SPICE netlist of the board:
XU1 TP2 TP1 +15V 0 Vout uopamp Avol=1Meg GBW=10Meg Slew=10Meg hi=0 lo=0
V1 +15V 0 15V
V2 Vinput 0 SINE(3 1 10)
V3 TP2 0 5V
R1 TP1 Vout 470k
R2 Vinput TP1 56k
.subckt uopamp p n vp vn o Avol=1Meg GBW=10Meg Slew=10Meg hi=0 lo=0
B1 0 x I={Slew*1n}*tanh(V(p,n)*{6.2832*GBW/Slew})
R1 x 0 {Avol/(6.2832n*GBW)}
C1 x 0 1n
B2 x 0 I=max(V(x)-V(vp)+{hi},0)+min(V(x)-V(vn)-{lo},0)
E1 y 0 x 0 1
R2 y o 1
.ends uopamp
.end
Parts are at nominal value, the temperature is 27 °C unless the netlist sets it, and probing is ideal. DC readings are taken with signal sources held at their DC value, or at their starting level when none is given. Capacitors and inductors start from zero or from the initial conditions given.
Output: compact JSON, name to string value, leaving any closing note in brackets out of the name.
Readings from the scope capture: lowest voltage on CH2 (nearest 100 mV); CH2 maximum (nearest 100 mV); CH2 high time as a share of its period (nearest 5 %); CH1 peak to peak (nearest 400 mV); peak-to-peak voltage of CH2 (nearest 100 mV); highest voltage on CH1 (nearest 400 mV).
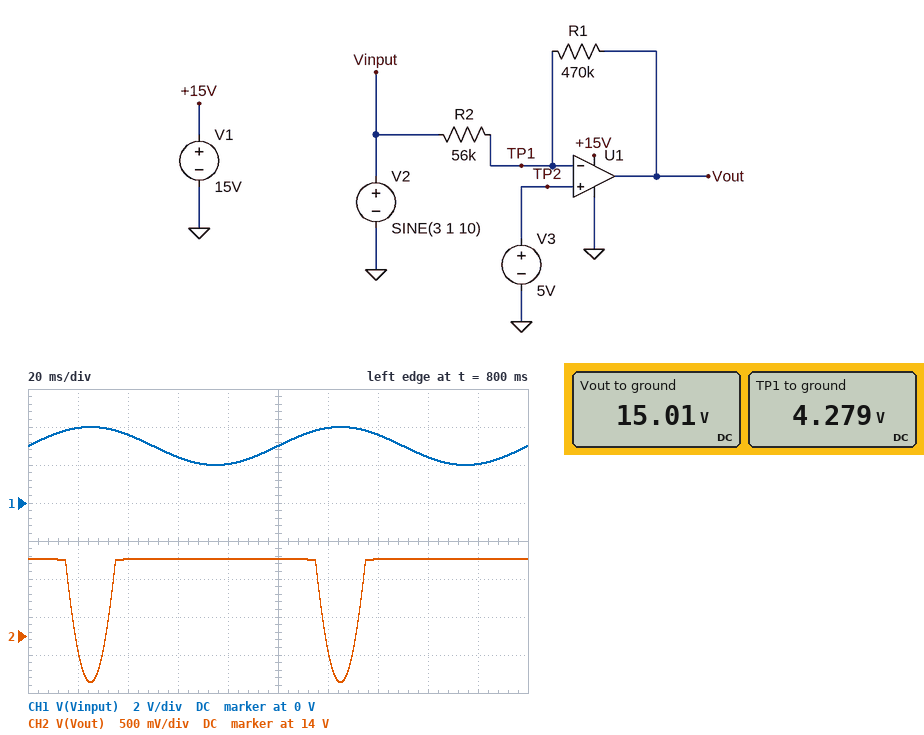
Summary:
{"lowest voltage on CH2": "13.4 V", "CH2 maximum": "15.0 V", "CH2 high time as a share of its period": "85 %", "CH1 peak to peak": "2.0 V", "peak-to-peak voltage of CH2": "1.6 V", "highest voltage on CH1": "4.0 V"}
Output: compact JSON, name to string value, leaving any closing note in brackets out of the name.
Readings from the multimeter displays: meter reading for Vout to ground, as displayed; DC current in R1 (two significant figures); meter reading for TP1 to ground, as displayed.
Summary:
{"meter reading for Vout to ground, as displayed": "15.01 V", "DC current in R1": "23 µA", "meter reading for TP1 to ground, as displayed": "4.279 V"}
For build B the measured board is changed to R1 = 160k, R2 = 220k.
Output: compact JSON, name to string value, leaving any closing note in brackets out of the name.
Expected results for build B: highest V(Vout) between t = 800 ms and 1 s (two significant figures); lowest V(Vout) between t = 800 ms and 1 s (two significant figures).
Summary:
{"highest V(Vout) between t = 800 ms and 1 s": "7.2 V", "lowest V(Vout) between t = 800 ms and 1 s": "5.7 V"}
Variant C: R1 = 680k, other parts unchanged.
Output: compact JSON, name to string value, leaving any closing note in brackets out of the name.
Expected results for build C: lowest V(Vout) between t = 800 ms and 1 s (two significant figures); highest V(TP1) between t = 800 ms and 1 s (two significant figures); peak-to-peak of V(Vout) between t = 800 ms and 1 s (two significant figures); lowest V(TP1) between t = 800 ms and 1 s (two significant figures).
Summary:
{"lowest V(Vout) between t = 800 ms and 1 s": "15 V", "highest V(TP1) between t = 800 ms and 1 s": "4.8 V", "peak-to-peak of V(Vout) between t = 800 ms and 1 s": "2.3 mV", "lowest V(TP1) between t = 800 ms and 1 s": "3.0 V"}
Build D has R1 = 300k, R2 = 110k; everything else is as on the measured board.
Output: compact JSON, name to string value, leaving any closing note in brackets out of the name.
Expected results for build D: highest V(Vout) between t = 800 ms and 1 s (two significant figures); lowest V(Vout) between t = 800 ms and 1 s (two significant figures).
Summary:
{"highest V(Vout) between t = 800 ms and 1 s": "13 V", "lowest V(Vout) between t = 800 ms and 1 s": "7.7 V"}
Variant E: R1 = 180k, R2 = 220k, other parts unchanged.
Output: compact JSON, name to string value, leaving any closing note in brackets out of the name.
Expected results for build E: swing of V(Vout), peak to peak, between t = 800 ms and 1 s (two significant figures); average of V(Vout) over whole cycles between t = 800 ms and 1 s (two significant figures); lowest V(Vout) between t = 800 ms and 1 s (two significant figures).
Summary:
{"swing of V(Vout), peak to peak, between t = 800 ms and 1 s": "1.6 V", "average of V(Vout) over whole cycles between t = 800 ms and 1 s": "6.6 V", "lowest V(Vout) between t = 800 ms and 1 s": "5.8 V"}
